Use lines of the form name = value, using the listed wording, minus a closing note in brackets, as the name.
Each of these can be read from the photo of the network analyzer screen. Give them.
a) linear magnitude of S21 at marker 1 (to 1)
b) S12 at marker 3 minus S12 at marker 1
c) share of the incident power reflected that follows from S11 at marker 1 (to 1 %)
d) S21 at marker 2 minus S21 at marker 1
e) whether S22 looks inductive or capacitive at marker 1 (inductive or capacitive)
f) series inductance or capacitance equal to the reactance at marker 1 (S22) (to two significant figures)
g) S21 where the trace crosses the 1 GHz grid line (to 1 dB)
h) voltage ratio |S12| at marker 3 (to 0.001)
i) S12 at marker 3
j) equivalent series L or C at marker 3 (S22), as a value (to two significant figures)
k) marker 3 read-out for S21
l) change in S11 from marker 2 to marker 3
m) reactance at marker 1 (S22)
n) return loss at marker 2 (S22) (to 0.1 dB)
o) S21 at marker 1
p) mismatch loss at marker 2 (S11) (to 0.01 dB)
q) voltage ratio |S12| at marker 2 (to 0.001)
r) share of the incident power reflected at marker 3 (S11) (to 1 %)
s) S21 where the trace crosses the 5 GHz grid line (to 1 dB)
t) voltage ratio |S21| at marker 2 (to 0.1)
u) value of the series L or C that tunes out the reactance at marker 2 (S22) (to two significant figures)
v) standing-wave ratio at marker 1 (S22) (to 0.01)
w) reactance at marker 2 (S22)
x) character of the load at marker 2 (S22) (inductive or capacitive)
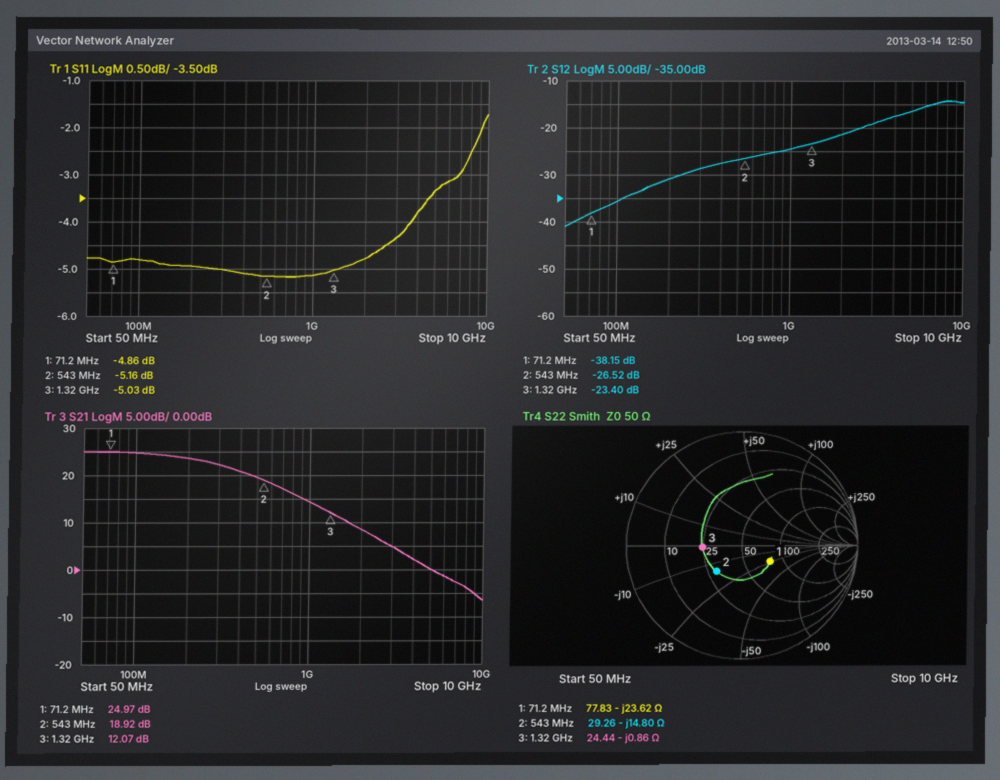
linear magnitude of S21 at marker 1 = 18
S12 at marker 3 minus S12 at marker 1 = 14.75 dB
share of the incident power reflected that follows from S11 at marker 1 = 33 %
S21 at marker 2 minus S21 at marker 1 = -6.05 dB
whether S22 looks inductive or capacitive at marker 1 = capacitive
series inductance or capacitance equal to the reactance at marker 1 (S22) = 95 pF
S21 where the trace crosses the 1 GHz grid line = 14 dB
voltage ratio |S12| at marker 3 = 0.068
S12 at marker 3 = -23.40 dB
equivalent series L or C at marker 3 (S22), as a value = 140 pF
marker 3 read-out for S21 = 12.07 dB
change in S11 from marker 2 to marker 3 = 0.13 dB
reactance at marker 1 = -23.62 Ω
return loss at marker 2 (S22) = 10.0 dB
S21 at marker 1 = 24.97 dB
mismatch loss at marker 2 (S11) = 1.58 dB
voltage ratio |S12| at marker 2 = 0.047
share of the incident power reflected at marker 3 (S11) = 31 %
S21 where the trace crosses the 5 GHz grid line = 0 dB
voltage ratio |S21| at marker 2 = 8.8
value of the series L or C that tunes out the reactance at marker 2 (S22) = 4.3 nH
standing-wave ratio at marker 1 (S22) = 1.78
reactance at marker 2 = -14.80 Ω
character of the load at marker 2 (S22) = capacitive
